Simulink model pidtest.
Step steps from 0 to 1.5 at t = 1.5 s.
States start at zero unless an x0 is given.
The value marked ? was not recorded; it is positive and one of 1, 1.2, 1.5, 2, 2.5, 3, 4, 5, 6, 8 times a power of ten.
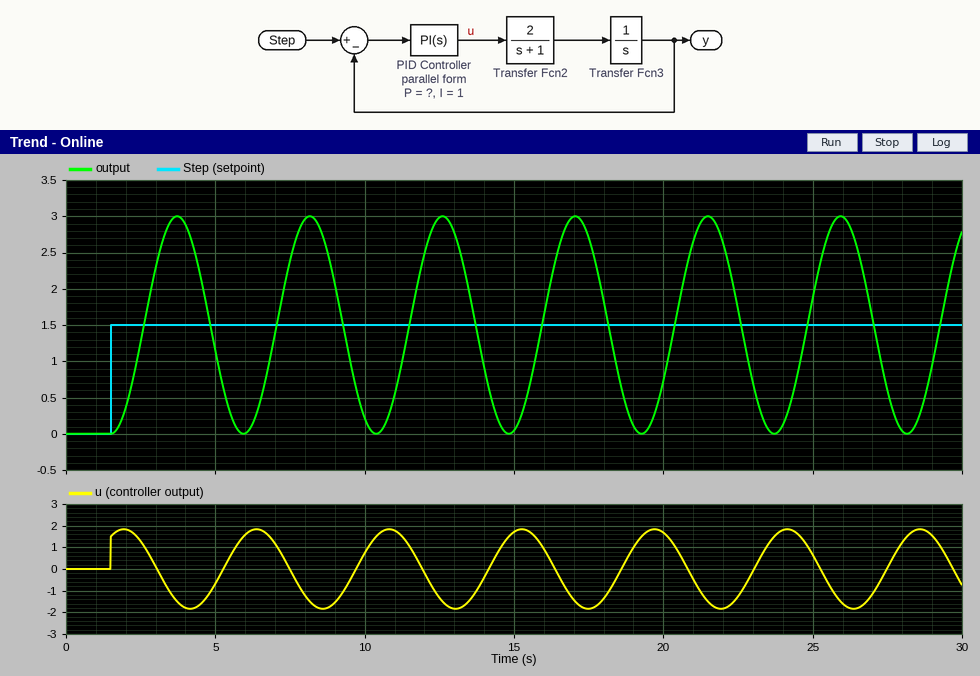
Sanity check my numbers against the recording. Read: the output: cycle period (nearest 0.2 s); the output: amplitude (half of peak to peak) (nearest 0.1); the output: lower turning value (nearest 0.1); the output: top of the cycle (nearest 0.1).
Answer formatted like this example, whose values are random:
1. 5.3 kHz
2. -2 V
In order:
1. 4.4 s
2. 1.5
3. 0.0
4. 3.0
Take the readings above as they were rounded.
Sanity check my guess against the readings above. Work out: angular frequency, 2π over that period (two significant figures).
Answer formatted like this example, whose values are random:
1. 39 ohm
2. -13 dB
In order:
1. 1.4 rad/s
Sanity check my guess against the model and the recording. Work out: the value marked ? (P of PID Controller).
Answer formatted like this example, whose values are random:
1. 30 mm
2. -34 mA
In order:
1. 1
